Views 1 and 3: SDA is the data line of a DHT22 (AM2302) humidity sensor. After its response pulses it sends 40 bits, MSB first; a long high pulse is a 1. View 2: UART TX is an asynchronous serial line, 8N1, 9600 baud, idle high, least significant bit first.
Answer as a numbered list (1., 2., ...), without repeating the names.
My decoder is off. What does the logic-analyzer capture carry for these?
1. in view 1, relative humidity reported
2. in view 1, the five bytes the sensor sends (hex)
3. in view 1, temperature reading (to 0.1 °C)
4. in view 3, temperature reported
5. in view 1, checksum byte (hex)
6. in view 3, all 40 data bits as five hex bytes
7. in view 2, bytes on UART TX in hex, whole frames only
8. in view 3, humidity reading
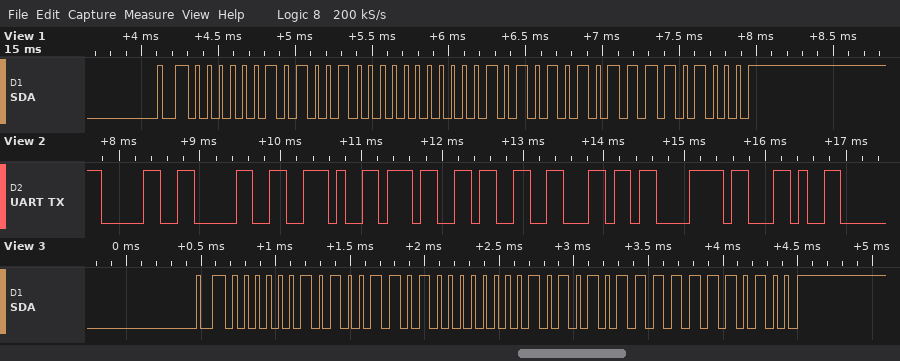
1. 65.6 %
2. 02 90 01 55 E8
3. 34.1 °C
4. 34.3 °C
5. 0xE8
6. 02 9A 01 57 F4
7. 30 30 2E 37 33 6C 78 2C
8. 66.6 %
